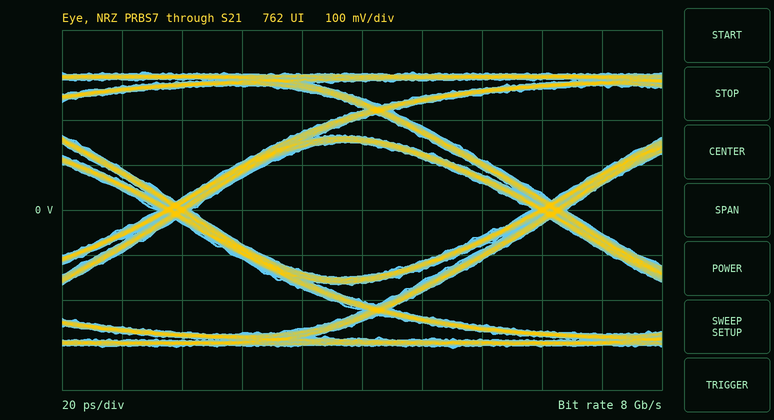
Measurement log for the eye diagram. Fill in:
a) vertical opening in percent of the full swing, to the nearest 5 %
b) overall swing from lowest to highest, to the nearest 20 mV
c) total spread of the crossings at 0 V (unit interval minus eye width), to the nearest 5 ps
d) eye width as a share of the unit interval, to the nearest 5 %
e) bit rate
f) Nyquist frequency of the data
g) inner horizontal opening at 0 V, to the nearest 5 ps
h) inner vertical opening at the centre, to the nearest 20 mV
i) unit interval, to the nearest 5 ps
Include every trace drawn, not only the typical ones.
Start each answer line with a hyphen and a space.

- 50 %
- 620 mV
- 10 ps
- 90 %
- 8 Gb/s
- 4 GHz
- 115 ps
- 300 mV
- 125 ps
